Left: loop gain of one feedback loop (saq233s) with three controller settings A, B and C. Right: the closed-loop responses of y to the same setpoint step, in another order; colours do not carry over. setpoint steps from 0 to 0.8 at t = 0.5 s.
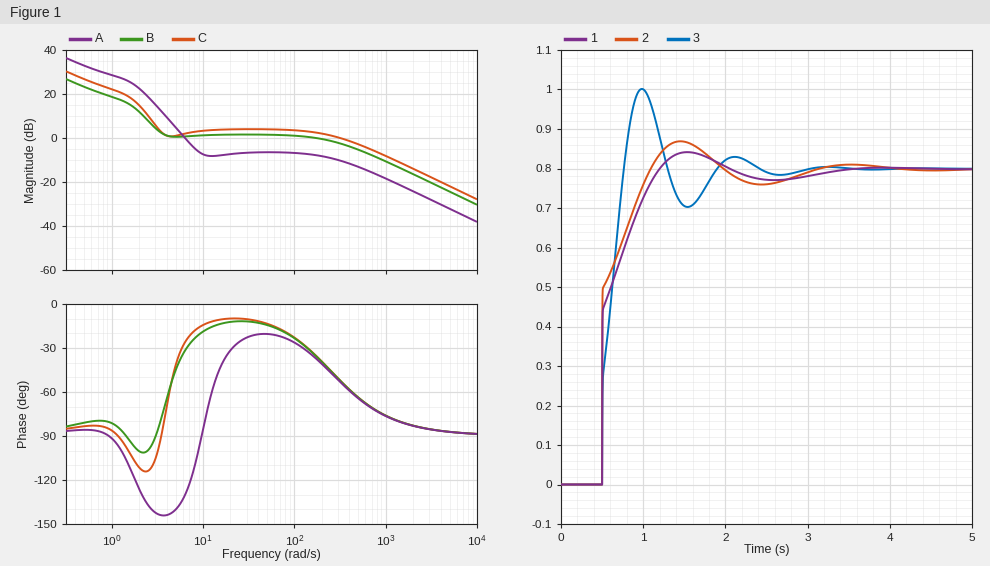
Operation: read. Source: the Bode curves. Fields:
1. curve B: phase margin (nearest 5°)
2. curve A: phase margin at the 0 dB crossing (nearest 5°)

145°
50°
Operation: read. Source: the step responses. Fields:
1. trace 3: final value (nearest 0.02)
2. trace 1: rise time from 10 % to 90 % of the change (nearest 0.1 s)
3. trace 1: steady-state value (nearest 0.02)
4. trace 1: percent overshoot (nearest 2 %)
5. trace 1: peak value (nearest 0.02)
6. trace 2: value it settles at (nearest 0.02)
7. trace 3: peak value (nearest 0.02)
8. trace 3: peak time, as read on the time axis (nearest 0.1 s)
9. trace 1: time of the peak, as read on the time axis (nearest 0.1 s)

0.80
0.5 s
0.80
6 %
0.84
0.80
1.00
1.0 s
1.5 s
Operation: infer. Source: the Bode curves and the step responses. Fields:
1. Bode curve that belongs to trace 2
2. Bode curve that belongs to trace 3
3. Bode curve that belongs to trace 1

C
A
B
